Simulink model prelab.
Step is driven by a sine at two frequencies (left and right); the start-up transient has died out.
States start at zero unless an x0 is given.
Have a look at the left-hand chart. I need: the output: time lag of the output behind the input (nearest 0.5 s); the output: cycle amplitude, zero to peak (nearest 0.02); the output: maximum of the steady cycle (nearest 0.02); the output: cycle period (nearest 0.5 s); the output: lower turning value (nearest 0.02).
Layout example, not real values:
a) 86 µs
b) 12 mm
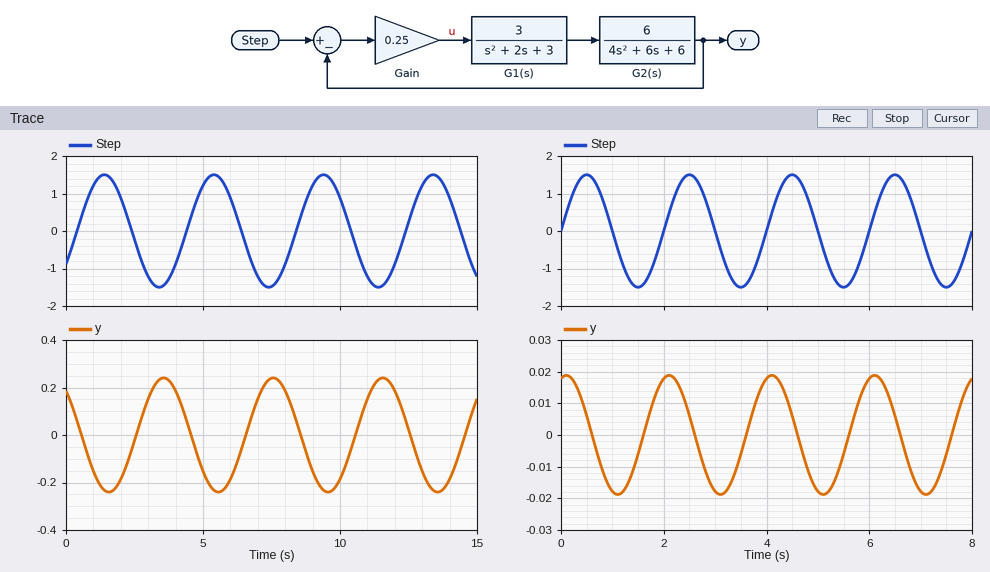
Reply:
a) 2.0 s
b) 0.24
c) 0.24
d) 4.0 s
e) -0.24
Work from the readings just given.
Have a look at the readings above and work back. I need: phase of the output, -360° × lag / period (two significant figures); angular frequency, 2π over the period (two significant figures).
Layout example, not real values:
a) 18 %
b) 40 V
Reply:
a) -180°
b) 1.6 rad/s
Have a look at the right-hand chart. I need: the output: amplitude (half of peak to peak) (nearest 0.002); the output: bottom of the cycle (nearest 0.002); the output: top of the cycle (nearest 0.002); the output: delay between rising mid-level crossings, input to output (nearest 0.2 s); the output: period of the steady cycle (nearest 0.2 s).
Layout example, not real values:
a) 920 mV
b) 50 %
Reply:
a) 0.018
b) -0.018
c) 0.018
d) 1.6 s
e) 2.0 s
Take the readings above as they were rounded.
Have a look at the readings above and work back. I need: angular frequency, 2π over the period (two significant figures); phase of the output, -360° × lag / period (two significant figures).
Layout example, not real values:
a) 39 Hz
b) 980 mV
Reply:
a) 3.1 rad/s
b) -290°
